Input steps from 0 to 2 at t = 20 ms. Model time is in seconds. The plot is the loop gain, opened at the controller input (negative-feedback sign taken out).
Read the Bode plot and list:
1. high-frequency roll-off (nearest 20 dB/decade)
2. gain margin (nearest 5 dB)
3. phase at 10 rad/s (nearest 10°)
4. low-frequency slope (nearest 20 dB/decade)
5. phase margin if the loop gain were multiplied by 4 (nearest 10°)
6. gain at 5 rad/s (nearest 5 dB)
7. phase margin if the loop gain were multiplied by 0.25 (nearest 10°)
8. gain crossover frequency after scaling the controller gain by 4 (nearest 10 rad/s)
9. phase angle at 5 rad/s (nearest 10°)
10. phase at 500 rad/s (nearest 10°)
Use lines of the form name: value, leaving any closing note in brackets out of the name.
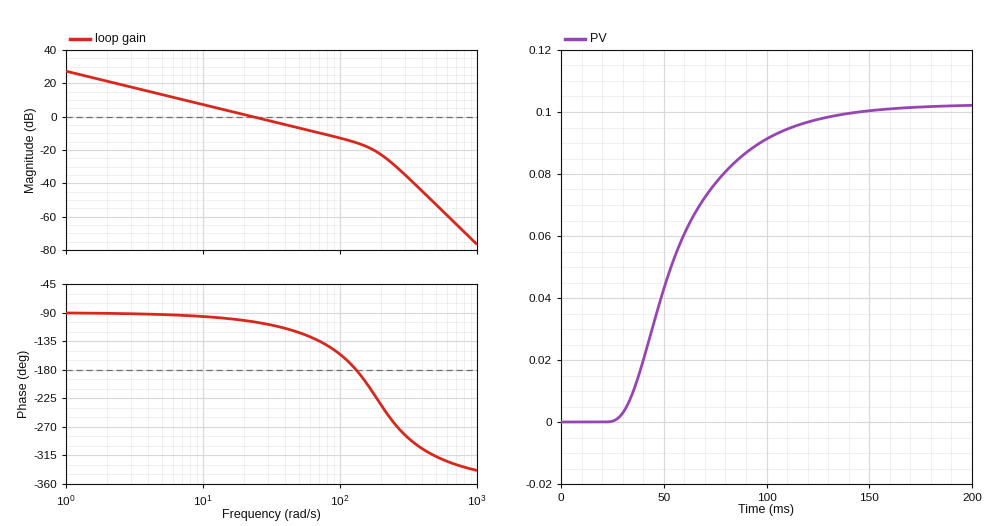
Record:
high-frequency roll-off: -80 dB/decade
gain margin: 15 dB
phase at 10 rad/s: -100°
low-frequency slope: -20 dB/decade
phase margin if the loop gain were multiplied by 4: 30°
gain at 5 rad/s: 15 dB
phase margin if the loop gain were multiplied by 0.25: 90°
gain crossover frequency after scaling the controller gain by 4: 90 rad/s
phase angle at 5 rad/s: -90°
phase at 500 rad/s: -320°
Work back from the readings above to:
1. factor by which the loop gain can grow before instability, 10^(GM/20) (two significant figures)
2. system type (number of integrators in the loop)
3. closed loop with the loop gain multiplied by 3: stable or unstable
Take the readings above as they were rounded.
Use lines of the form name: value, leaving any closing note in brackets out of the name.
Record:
factor by which the loop gain can grow before instability, 10^(GM/20): 5.6
system type: 1
closed loop with the loop gain multiplied by 3: stable or unstable: stable
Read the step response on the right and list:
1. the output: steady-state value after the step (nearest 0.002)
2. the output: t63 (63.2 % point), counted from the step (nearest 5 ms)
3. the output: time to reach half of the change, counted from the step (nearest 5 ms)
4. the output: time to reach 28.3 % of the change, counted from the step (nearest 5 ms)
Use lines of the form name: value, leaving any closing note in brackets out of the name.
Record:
the output: steady-state value after the step: 0.102
the output: t63 (63.2 % point), counted from the step: 45 ms
the output: time to reach half of the change, counted from the step: 35 ms
the output: time to reach 28.3 % of the change, counted from the step: 25 ms
